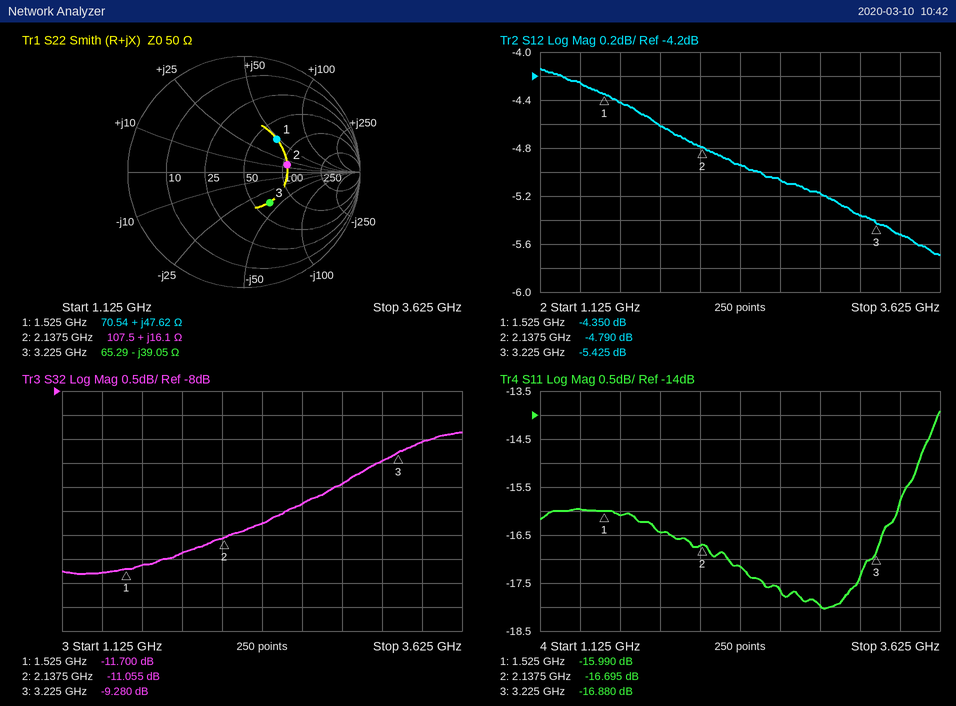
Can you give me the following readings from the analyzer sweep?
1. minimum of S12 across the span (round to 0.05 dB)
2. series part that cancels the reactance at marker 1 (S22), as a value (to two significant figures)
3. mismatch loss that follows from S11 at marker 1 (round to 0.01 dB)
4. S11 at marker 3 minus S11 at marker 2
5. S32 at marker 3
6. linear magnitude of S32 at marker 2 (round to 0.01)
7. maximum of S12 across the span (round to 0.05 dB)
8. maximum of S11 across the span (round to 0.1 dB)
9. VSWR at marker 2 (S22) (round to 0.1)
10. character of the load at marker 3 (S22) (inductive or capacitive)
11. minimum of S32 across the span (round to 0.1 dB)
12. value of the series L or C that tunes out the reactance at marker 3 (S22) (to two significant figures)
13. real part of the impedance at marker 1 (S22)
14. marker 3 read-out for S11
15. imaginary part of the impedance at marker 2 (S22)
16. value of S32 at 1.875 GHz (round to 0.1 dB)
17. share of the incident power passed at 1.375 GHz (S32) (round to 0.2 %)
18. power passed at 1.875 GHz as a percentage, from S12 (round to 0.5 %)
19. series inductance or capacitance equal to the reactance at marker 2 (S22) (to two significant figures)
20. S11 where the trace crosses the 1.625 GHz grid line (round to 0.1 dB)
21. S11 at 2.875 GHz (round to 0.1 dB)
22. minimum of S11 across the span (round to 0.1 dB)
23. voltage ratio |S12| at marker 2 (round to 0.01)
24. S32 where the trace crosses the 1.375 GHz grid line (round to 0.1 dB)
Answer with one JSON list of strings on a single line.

["-5.70 dB", "2.2 pF", "0.11 dB", "-0.185 dB", "-9.280 dB", "0.28", "-4.15 dB", "-13.9 dB", "2.2", "capacitive", "-11.8 dB", "1.9 nH", "70.54 Ω", "-16.880 dB", "+16.1 Ω", "-11.4 dB", "6.6 %", "34.5 %", "1.2 nH", "-16.1 dB", "-18.0 dB", "-18.0 dB", "0.58", "-11.8 dB"]
